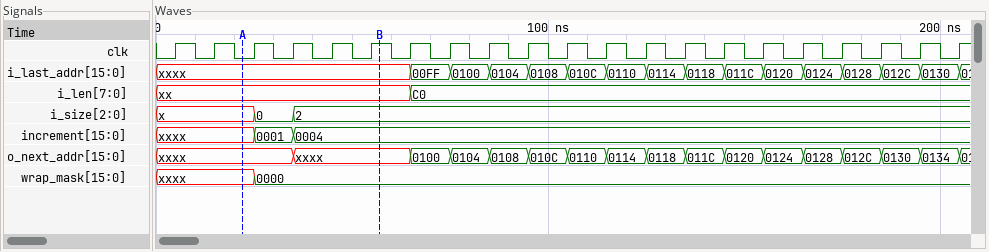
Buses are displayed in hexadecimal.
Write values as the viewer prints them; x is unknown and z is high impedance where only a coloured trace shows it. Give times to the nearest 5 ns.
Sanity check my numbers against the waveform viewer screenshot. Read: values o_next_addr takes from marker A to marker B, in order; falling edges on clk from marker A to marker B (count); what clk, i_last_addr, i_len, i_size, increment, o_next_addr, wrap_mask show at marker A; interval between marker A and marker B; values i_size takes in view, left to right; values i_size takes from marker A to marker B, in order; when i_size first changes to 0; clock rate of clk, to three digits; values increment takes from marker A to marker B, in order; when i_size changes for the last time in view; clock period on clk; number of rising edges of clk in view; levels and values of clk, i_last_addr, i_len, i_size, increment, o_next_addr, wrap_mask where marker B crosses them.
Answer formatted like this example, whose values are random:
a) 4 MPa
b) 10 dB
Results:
a) xxxx, xxxx
b) 3
c) clk=0, i_last_addr=xxxx, i_len=xx, i_size=x, increment=xxxx, o_next_addr=xxxx, wrap_mask=xxxx
d) 35 ns
e) x, 0, 2
f) x, 0, 2
g) 25 ns
h) 100 MHz
i) xxxx, 0001, 0004
j) 35 ns
k) 10 ns
l) 21
m) clk=1, i_last_addr=xxxx, i_len=xx, i_size=2, increment=0004, o_next_addr=xxxx, wrap_mask=0000
